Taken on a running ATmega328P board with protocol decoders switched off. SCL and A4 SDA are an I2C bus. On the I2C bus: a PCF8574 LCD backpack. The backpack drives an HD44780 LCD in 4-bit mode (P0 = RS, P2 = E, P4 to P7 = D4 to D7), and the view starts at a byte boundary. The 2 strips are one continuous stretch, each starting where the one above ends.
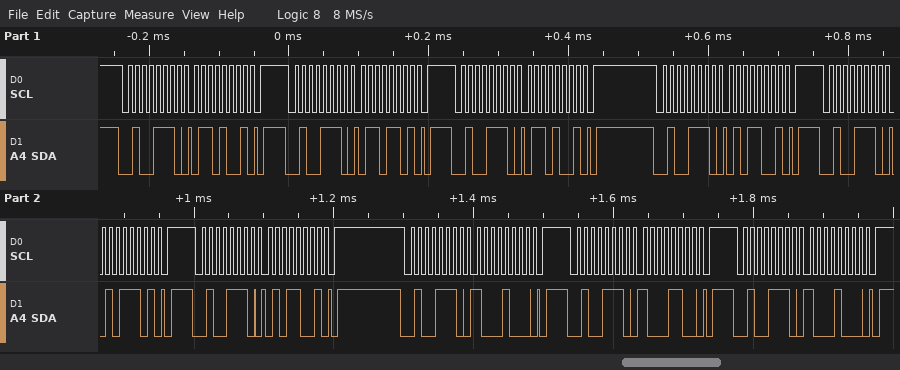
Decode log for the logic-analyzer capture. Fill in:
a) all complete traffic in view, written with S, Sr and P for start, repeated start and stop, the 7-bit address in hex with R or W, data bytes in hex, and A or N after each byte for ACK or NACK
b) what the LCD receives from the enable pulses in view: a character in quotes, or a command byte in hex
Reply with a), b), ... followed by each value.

a) S 27W A 69 A P S 27W A 6D A P S 27W A 69 A P S 27W A 59 A P S 27W A 5D A P S 27W A 59 A P S 27W A 88 A P S 27W A 8C A P S 27W A 88 A P
b) 'e'
